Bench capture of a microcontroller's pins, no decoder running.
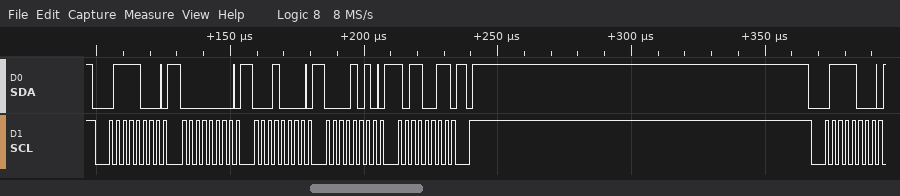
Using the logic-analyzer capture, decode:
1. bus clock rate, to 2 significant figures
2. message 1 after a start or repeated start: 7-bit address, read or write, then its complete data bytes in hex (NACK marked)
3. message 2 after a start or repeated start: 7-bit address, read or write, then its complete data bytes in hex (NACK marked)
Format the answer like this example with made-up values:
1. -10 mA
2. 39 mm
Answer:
1. 400 kHz
2. 0x3C write: 00 10 0A B3
3. 0x3C write
